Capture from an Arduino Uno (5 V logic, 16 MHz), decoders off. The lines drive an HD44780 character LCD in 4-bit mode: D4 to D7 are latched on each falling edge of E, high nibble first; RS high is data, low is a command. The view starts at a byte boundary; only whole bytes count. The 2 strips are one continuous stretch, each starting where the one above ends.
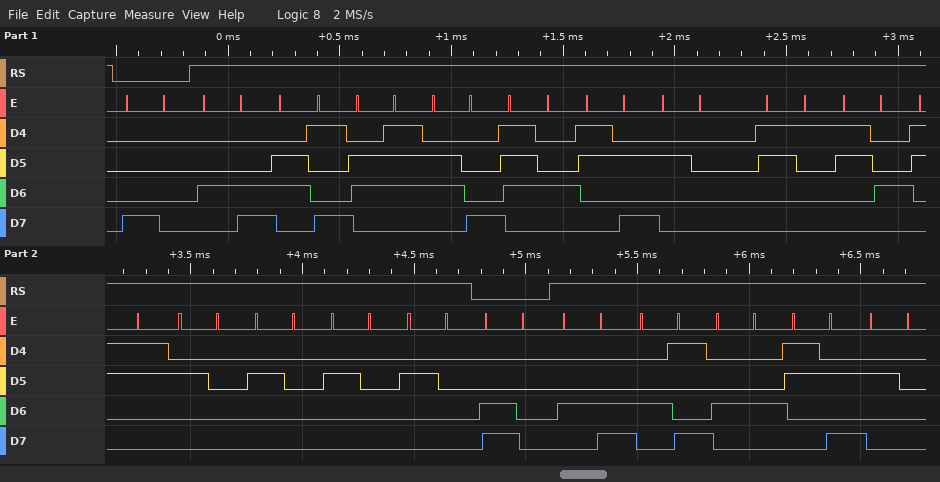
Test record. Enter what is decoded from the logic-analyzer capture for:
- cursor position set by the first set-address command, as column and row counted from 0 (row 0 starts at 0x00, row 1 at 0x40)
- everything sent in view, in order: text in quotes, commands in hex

column 0, row 0
0x80 "Light: 143    " 0xC0 "LID: "
